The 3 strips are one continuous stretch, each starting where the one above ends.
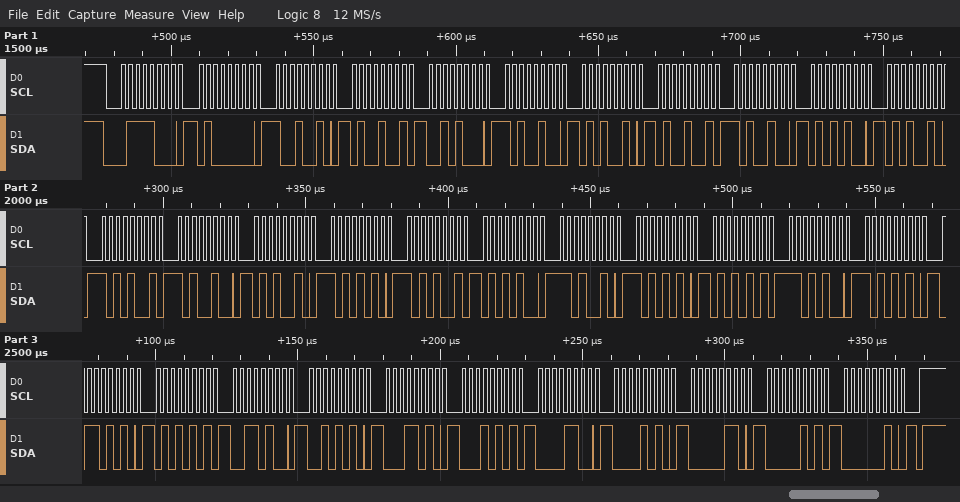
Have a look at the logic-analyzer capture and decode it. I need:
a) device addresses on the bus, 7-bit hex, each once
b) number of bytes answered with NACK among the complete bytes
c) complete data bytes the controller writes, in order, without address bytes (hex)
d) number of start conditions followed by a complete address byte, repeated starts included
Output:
0x3C
0
40 92 49 28 A4 52 49 A4 54 52 A9 A4 52 AA A9 54 D2 AA 55 D4 AA 6A 55 34 2A 1A 15 0C 0A 06 05 02
1
